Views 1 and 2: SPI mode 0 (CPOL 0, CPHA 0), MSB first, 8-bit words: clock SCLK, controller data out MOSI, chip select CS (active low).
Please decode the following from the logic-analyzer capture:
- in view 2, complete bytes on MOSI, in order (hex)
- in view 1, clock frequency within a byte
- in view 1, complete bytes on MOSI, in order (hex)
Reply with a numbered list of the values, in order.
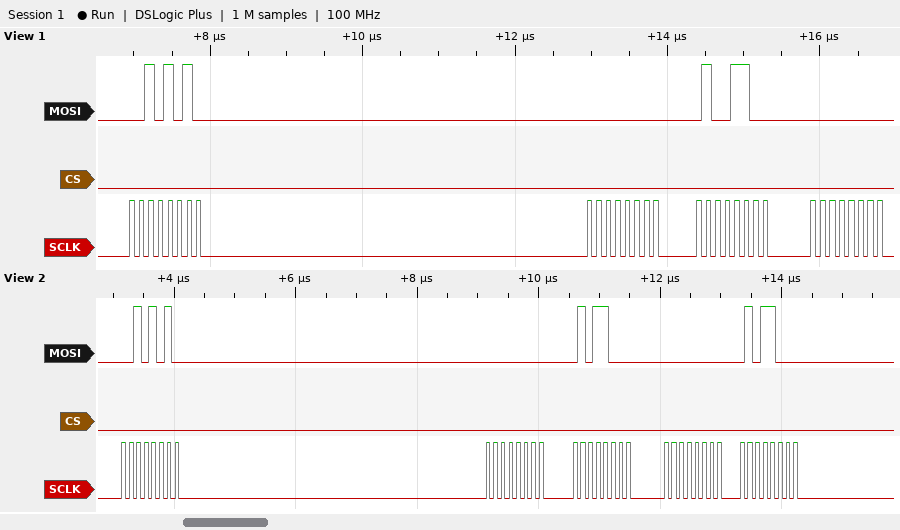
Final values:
1. 0x2A 0x00 0x58 0x00 0x58
2. 8 MHz
3. 2A 00 4C 00
